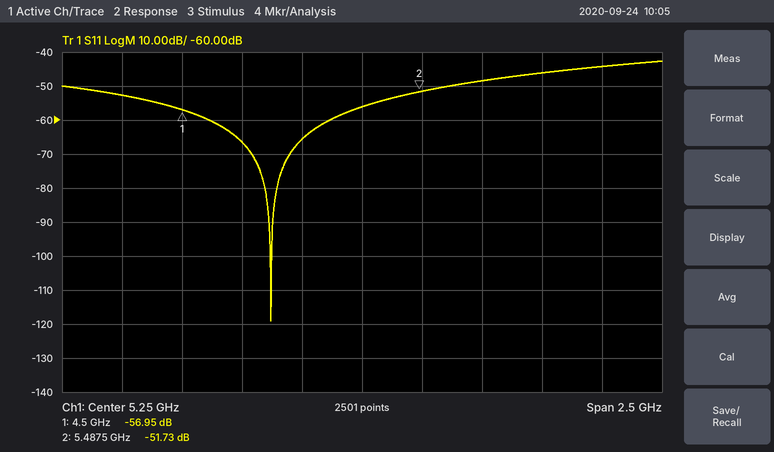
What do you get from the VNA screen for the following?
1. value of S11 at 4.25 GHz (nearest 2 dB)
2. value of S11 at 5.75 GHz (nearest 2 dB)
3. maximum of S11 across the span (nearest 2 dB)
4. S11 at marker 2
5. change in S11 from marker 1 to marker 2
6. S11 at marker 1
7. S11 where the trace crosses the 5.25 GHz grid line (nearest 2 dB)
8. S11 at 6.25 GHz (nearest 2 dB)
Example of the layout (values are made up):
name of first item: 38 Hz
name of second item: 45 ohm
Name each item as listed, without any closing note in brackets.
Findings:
value of S11 at 4.25 GHz: -52 dB
value of S11 at 5.75 GHz: -48 dB
maximum of S11 across the span: -42 dB
S11 at marker 2: -51.73 dB
change in S11 from marker 1 to marker 2: 5.22 dB
S11 at marker 1: -56.95 dB
S11 where the trace crosses the 5.25 GHz grid line: -56 dB
S11 at 6.25 GHz: -44 dB
